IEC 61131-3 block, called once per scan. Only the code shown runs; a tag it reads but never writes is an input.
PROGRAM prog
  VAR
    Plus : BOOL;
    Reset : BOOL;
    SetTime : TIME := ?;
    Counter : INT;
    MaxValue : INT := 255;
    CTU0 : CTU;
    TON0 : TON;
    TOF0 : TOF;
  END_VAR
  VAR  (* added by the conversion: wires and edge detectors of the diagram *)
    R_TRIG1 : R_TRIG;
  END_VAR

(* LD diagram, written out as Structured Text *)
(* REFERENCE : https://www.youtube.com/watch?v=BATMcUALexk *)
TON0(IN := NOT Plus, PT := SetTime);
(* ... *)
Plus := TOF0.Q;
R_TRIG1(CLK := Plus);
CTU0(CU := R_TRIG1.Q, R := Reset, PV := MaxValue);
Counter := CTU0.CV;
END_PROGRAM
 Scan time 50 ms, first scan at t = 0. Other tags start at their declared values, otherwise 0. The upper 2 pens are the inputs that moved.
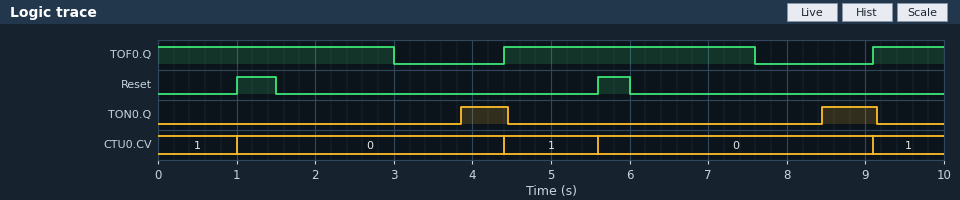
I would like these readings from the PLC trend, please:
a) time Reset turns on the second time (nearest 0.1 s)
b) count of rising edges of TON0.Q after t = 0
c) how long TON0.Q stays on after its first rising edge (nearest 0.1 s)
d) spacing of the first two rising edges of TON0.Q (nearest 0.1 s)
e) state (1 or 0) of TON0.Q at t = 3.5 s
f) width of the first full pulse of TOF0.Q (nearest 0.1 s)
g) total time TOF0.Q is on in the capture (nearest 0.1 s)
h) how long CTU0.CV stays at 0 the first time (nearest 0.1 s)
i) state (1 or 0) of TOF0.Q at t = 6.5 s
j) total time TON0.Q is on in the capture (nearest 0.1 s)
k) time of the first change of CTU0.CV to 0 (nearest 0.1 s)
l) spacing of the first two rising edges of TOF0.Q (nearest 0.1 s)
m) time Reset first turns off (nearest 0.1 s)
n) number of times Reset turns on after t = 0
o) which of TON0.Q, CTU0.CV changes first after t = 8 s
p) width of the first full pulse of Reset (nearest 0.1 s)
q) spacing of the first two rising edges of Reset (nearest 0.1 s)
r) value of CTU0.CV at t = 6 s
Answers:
5.6 s
2
0.6 s
4.6 s
0
3.2 s
7.1 s
3.4 s
1
1.3 s
1.0 s
4.7 s
1.5 s
2
TON0.Q
0.5 s
4.6 s
0
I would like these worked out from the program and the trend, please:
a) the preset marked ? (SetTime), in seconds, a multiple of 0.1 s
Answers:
0.8 s
